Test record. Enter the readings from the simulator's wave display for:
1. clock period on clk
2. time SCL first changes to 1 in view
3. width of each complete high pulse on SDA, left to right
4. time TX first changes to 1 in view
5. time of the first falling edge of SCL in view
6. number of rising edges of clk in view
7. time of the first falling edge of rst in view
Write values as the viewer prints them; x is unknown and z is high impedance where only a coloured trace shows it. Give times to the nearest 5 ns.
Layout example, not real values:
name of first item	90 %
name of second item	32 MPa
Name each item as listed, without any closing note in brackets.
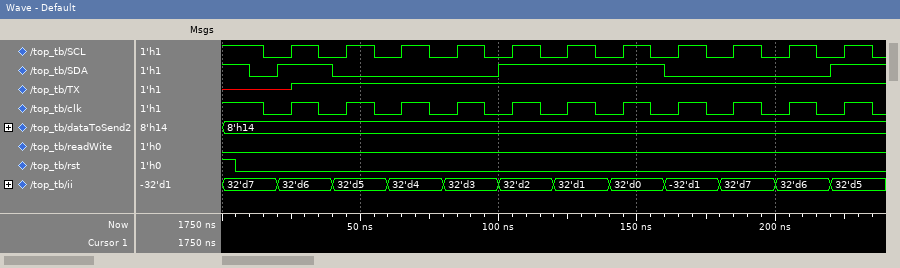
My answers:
clock period on clk	20 ns
time SCL first changes to 1 in view	25 ns
width of each complete high pulse on SDA, left to right	20 ns, 60 ns
time TX first changes to 1 in view	25 ns
time of the first falling edge of SCL in view	15 ns
number of rising edges of clk in view	11
time of the first falling edge of rst in view	5 ns
